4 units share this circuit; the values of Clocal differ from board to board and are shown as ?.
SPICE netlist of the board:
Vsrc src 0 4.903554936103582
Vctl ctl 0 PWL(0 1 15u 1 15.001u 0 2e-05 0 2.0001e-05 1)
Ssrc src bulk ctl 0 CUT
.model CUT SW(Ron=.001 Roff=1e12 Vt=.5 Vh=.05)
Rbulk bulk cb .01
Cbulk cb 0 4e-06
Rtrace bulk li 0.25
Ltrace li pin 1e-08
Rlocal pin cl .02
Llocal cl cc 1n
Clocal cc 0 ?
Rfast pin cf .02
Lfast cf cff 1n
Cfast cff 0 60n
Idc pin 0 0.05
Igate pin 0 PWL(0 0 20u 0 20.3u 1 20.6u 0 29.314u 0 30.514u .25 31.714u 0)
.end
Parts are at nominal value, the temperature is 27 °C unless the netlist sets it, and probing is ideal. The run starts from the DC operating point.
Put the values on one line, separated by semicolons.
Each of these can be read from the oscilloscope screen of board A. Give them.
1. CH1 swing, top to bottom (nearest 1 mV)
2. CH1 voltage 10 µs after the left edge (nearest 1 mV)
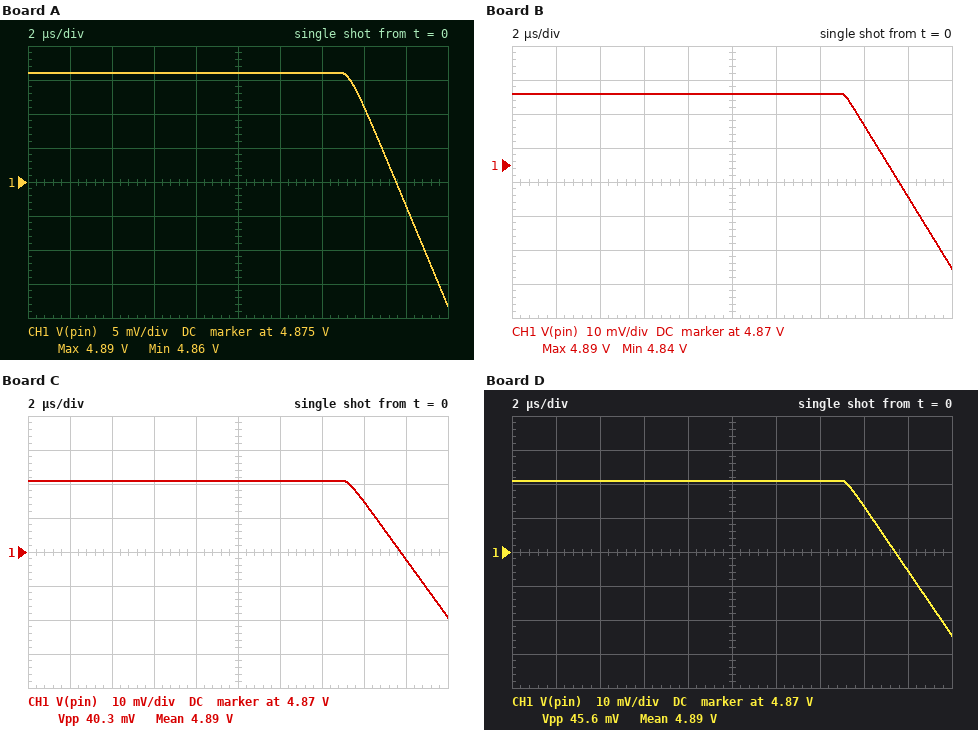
34 mV; 4.891 V
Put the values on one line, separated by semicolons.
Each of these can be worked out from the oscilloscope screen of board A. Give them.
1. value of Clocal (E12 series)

2.7 µF
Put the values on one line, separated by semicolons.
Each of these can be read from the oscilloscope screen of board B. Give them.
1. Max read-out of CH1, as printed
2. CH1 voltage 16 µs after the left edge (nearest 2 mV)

4.89 V; 4.882 V
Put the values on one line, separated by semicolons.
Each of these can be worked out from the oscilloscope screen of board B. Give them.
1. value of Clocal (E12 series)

680 nF
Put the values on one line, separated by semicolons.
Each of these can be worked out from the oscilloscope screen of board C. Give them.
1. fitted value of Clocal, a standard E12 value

1.8 µF
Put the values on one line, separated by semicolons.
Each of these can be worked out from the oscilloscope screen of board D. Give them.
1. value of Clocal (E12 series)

1.2 µF
